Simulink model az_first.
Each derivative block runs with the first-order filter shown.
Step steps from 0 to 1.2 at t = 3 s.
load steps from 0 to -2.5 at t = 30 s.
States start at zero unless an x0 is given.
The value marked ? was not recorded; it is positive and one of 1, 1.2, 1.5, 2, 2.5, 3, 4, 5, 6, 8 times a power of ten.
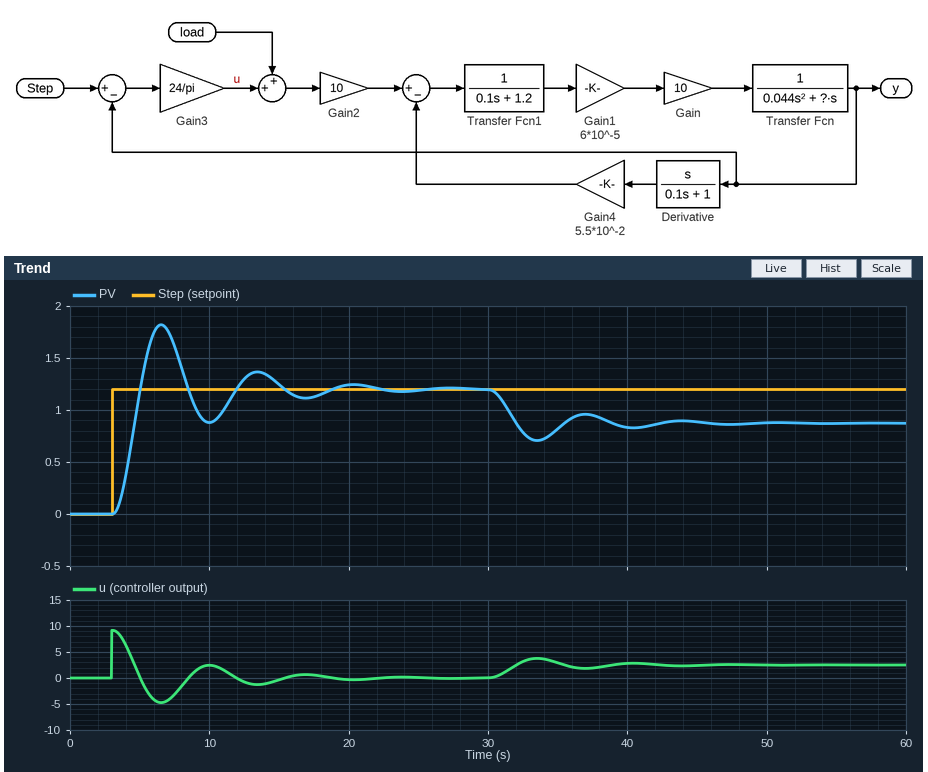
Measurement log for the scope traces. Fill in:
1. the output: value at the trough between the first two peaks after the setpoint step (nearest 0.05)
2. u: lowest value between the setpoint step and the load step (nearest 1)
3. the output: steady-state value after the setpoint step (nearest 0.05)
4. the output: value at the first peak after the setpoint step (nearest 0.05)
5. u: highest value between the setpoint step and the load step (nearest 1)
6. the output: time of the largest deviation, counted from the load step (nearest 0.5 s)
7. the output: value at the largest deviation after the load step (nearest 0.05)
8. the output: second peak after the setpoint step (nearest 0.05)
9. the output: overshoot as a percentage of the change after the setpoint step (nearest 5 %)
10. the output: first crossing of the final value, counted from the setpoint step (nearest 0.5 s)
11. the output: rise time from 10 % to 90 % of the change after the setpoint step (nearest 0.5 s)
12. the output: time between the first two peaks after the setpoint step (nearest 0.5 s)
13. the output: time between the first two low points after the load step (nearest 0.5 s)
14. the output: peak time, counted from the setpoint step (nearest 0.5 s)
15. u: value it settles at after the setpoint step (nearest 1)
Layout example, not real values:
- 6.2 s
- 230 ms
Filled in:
- 0.90
- -5
- 1.20
- 1.80
- 9
- 3.5 s
- 0.70
- 1.35
- 50 %
- 2.0 s
- 1.5 s
- 7.0 s
- 7.0 s
- 3.5 s
- 0
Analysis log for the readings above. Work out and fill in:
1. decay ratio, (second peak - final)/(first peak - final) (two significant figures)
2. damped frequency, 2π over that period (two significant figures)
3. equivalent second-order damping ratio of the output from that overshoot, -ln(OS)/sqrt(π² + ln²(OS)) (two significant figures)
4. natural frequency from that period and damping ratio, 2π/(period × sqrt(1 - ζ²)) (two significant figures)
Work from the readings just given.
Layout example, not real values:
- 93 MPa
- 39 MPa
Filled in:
- 0.25
- 0.90 rad/s
- 0.22
- 0.92 rad/s
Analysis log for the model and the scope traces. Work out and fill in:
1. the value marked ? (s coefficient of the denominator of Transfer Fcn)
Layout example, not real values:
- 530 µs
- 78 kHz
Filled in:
- 0.02
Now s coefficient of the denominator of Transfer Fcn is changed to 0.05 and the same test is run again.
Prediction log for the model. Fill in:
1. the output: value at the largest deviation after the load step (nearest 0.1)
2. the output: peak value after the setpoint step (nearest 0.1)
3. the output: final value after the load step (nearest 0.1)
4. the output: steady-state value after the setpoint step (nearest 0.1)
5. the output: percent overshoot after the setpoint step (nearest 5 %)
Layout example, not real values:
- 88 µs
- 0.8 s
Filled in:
- 0.8
- 1.3
- 0.9
- 1.2
- 10 %
